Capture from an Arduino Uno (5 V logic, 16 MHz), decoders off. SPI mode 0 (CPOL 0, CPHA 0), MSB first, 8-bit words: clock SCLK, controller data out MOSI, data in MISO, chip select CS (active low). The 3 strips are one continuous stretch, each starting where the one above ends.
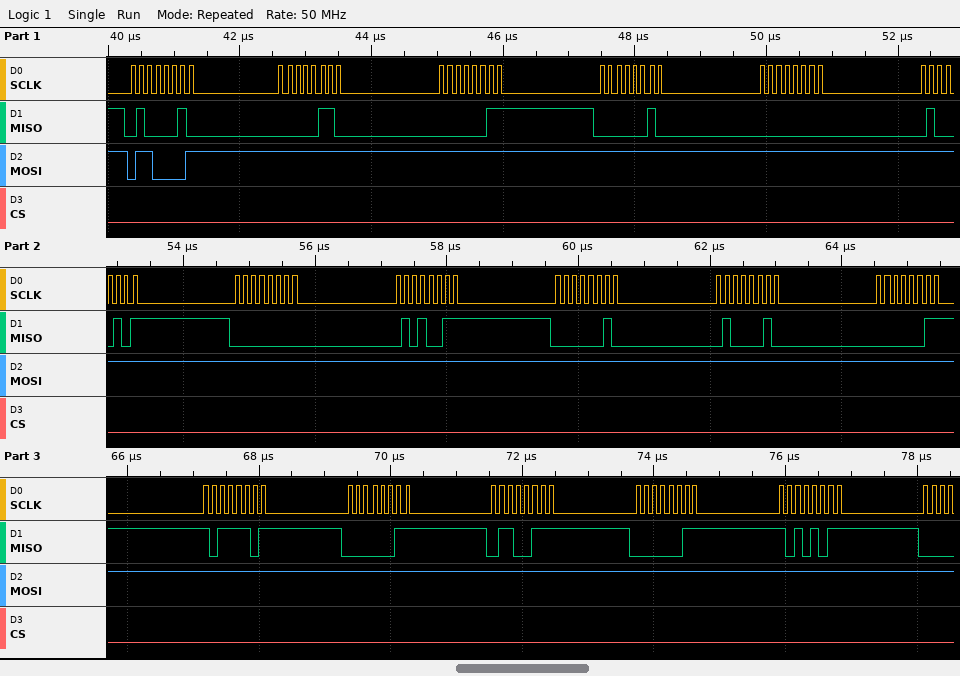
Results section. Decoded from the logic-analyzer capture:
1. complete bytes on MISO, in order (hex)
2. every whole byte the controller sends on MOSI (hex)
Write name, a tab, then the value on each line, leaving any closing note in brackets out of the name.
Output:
complete bytes on MISO, in order	0x42 0x06 0x03 0x02 0x00 0x45 0x00 0x53 0x02 0x42 0x03 0xBD 0x03 0x67 0x03 0xAB
every whole byte the controller sends on MOSI	0x61 0xFF 0xFF 0xFF 0xFF 0xFF 0xFF 0xFF 0xFF 0xFF 0xFF 0xFF 0xFF 0xFF 0xFF 0xFF
